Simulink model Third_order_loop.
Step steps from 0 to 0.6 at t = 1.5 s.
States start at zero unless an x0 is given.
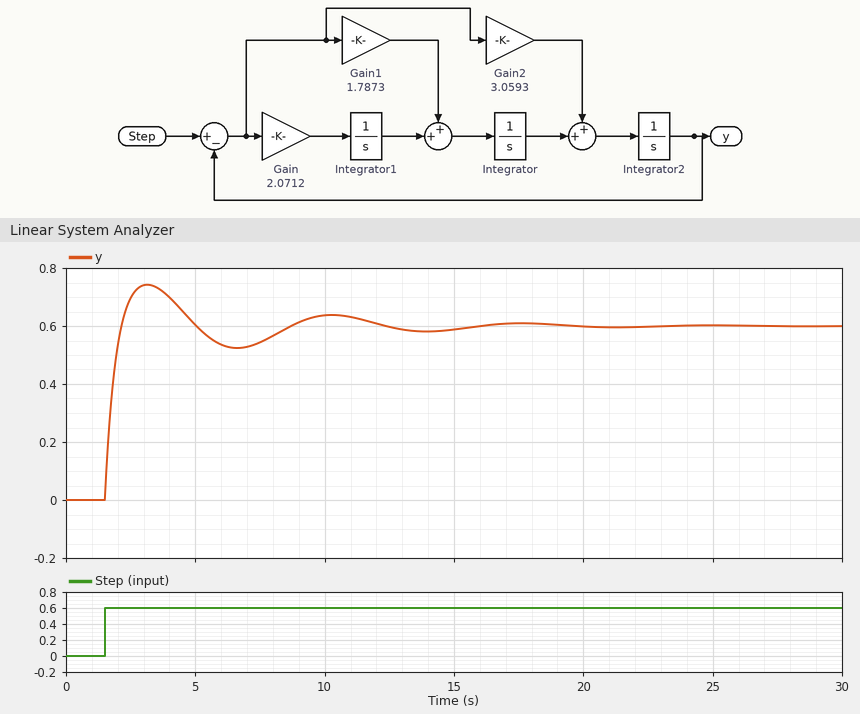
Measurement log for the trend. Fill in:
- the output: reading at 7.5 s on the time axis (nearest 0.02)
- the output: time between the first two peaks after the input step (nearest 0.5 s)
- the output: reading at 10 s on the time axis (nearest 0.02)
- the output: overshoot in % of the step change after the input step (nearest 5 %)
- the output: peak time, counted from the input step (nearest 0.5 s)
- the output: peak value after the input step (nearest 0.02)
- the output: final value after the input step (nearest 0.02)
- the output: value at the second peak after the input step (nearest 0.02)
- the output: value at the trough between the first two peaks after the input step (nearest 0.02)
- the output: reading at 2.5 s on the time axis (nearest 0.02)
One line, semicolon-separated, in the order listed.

0.54; 7.0 s; 0.64; 25 %; 1.5 s; 0.74; 0.60; 0.64; 0.52; 0.70
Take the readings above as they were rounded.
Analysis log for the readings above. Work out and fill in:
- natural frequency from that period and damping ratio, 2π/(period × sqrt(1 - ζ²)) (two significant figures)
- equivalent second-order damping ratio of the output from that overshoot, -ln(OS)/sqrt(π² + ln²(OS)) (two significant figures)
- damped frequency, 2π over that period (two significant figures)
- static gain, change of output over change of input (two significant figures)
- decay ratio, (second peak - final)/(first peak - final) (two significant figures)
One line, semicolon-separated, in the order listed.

0.98 rad/s; 0.40; 0.90 rad/s; 1.0; 0.29
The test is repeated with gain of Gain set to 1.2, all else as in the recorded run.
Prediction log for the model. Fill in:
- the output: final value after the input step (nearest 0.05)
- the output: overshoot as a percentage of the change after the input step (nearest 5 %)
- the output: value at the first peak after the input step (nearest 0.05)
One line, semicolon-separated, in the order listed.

0.60; 20 %; 0.70
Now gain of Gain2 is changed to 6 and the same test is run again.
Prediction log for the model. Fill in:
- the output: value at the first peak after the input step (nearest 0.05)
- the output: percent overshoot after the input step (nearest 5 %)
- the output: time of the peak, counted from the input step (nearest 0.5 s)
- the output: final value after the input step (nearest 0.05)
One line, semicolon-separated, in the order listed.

0.65; 10 %; 2.0 s; 0.60
